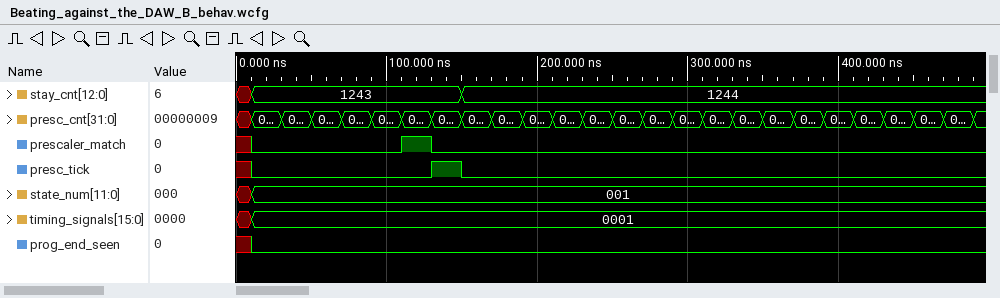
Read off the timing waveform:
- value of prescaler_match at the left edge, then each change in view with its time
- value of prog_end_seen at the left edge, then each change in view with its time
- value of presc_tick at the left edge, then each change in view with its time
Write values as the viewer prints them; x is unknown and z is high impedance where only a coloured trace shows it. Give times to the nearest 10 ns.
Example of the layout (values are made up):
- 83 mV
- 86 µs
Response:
- x, 0 at 10 ns, 1 at 110 ns, 0 at 130 ns
- x, 0 at 10 ns
- x, 0 at 10 ns, 1 at 130 ns, 0 at 150 ns
